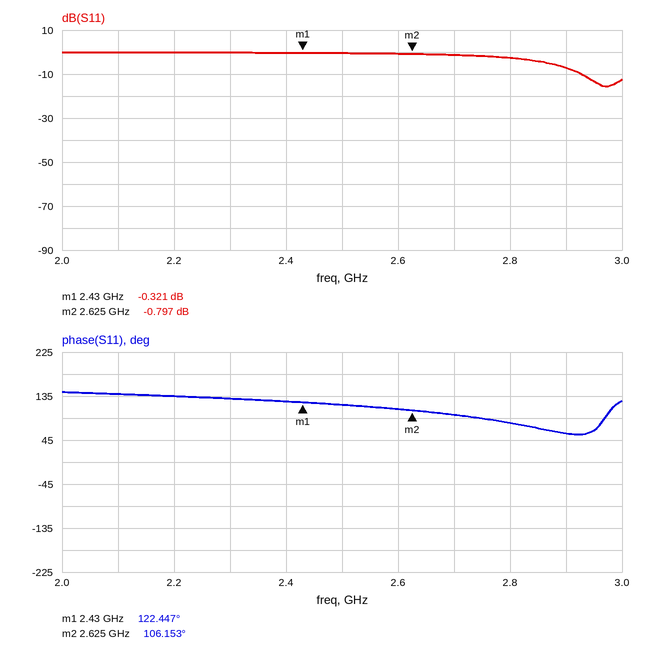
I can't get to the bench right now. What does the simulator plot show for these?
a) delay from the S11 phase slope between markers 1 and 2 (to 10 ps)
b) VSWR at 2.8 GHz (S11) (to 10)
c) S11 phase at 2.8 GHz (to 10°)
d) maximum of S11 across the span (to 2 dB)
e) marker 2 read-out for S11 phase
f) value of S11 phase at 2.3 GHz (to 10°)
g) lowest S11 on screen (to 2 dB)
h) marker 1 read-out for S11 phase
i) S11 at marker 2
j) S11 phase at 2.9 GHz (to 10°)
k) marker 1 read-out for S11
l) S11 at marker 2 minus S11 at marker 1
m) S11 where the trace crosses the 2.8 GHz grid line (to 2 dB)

230 ps
10
80°
0 dB
106.153°
130°
-16 dB
122.447°
-0.797 dB
60°
-0.321 dB
-0.476 dB
-2 dB
